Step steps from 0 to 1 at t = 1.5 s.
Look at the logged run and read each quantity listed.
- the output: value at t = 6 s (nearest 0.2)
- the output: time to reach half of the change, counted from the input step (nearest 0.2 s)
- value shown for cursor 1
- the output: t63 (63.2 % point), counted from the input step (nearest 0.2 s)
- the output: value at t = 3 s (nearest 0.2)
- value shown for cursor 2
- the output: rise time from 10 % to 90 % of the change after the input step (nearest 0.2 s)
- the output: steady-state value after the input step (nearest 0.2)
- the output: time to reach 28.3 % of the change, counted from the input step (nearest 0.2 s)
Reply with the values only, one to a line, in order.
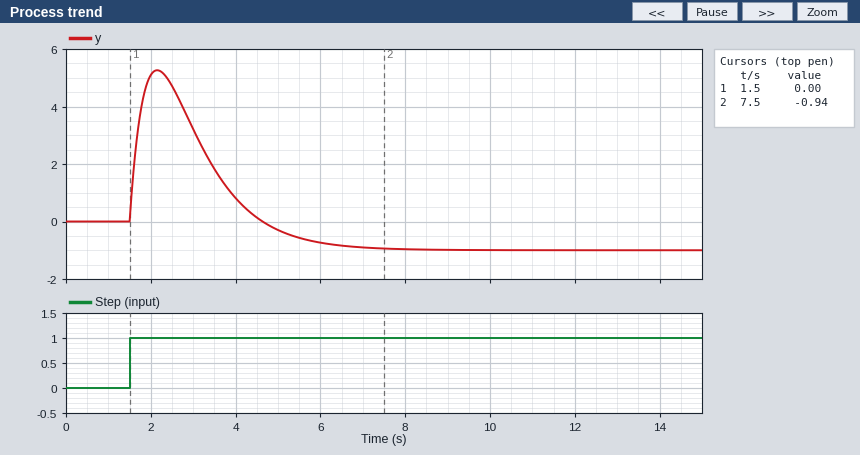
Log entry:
-0.8
3.8 s
0.00
4.2 s
3.2
-0.94
2.2 s
-1.0
3.4 s
